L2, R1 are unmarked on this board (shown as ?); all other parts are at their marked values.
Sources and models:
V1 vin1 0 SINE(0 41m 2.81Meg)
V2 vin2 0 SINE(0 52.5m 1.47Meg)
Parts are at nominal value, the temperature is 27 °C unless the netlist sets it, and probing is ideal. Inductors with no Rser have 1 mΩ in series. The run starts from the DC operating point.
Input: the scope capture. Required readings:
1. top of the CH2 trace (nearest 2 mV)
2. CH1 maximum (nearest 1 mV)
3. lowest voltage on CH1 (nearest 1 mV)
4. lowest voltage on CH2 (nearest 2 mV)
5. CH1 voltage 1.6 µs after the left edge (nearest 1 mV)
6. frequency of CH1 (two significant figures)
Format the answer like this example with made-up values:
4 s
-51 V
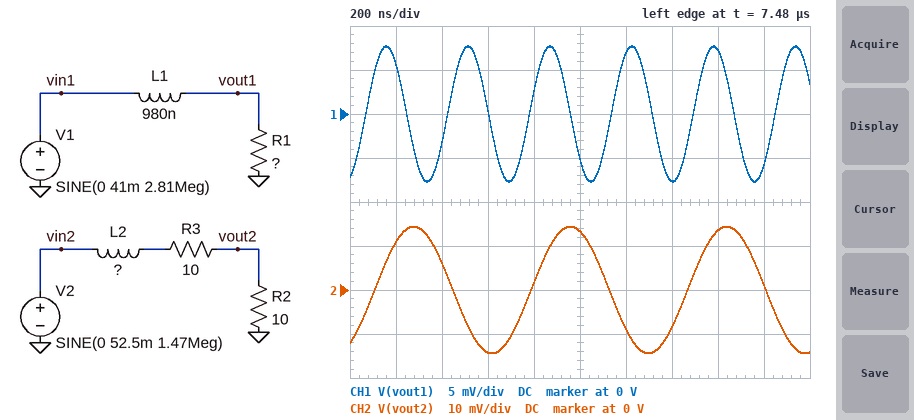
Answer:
14 mV
8 mV
-8 mV
-14 mV
7 mV
2.8 MHz
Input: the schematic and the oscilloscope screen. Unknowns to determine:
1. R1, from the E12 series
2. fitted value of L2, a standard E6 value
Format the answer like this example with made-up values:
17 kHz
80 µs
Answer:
3.3 Ω
3.3 µH
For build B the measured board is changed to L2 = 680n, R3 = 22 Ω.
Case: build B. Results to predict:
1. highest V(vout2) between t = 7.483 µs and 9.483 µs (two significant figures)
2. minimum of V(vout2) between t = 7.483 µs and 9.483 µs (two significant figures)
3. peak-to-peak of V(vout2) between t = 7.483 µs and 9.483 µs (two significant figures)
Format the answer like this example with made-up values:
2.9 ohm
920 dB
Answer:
16 mV
-16 mV
32 mV
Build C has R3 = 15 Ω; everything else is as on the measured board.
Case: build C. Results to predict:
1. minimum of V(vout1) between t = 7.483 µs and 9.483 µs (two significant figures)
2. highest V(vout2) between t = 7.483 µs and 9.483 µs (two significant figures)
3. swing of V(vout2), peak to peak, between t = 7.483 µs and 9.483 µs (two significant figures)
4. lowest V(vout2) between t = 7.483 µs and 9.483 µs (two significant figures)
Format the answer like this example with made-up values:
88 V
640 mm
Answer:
-7.7 mV
13 mV
27 mV
-13 mV
